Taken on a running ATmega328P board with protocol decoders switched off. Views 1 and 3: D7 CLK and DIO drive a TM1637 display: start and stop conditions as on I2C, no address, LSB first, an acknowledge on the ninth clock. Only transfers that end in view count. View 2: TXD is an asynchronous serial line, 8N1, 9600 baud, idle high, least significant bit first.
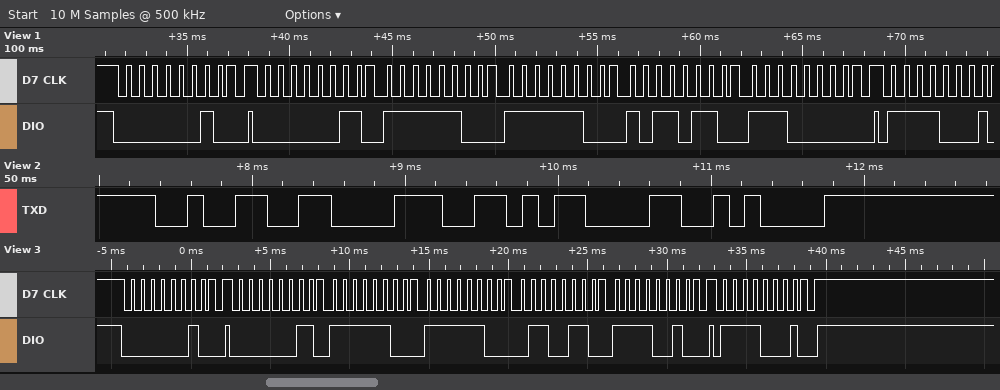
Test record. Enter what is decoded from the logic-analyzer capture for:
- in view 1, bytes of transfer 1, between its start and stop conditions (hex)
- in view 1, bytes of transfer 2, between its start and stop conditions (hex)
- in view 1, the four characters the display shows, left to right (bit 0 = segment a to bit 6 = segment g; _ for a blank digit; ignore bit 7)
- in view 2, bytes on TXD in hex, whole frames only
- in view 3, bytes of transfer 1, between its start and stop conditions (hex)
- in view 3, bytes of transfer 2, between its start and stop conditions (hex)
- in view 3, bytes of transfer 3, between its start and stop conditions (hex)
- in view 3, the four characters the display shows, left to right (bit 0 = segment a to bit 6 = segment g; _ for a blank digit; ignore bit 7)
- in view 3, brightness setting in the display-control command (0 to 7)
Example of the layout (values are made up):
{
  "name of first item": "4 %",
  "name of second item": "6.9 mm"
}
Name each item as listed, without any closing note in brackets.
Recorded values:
{
  "in view 1, bytes of transfer 1, between its start and stop conditions": "40",
  "in view 1, bytes of transfer 2, between its start and stop conditions": "C0 3F 3F 6D 07",
  "in view 1, the four characters the display shows, left to right": "0057",
  "in view 2, bytes on TXD in hex, whole frames only": "32 38 0D 0A",
  "in view 3, bytes of transfer 1, between its start and stop conditions": "40",
  "in view 3, bytes of transfer 2, between its start and stop conditions": "C0 3F 3F 66 4F",
  "in view 3, bytes of transfer 3, between its start and stop conditions": "8F",
  "in view 3, the four characters the display shows, left to right": "0043",
  "in view 3, brightness setting in the display-control command": "7"
}
